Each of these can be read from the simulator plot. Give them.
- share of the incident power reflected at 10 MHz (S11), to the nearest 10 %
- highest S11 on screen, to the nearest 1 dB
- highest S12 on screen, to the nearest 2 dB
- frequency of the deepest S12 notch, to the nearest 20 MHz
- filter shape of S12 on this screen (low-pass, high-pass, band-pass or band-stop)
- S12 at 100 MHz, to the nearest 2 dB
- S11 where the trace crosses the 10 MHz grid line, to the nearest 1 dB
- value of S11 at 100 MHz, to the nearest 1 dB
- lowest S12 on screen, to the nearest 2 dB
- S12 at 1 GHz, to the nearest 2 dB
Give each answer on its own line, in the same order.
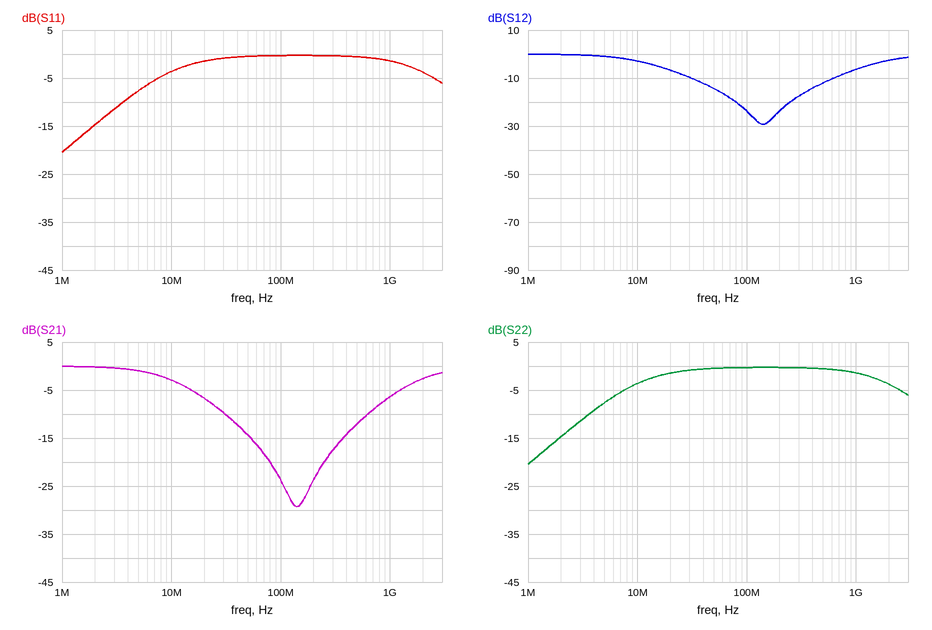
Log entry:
40 %
0 dB
0 dB
140 MHz
band-stop
-24 dB
-4 dB
0 dB
-30 dB
-6 dB
